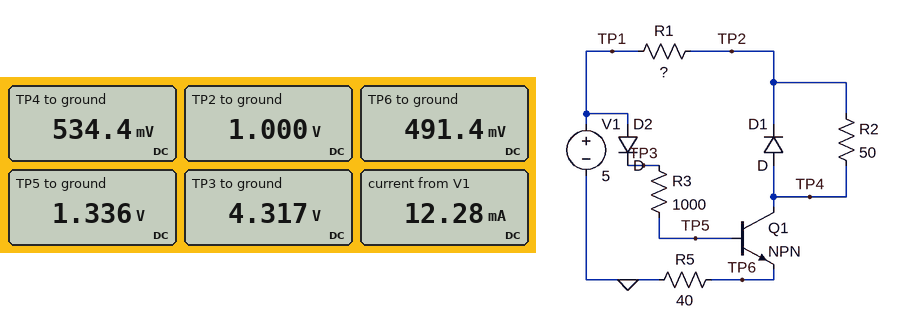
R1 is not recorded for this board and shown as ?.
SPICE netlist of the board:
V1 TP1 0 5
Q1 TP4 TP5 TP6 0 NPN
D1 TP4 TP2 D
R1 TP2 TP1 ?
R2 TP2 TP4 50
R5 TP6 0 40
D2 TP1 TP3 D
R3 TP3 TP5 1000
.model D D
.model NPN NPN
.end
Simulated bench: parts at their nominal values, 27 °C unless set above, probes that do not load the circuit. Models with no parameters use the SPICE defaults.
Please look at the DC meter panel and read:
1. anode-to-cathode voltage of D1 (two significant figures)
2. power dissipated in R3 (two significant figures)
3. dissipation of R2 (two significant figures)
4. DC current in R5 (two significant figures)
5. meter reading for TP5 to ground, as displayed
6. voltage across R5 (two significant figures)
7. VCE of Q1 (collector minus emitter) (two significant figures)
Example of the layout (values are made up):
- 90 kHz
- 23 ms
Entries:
- -470 mV
- 8.9 mW
- 4.3 mW
- 12 mA
- 1.336 V
- 490 mV
- 43 mV
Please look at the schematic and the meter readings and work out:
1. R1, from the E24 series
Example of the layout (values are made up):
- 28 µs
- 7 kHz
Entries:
- 430 Ω
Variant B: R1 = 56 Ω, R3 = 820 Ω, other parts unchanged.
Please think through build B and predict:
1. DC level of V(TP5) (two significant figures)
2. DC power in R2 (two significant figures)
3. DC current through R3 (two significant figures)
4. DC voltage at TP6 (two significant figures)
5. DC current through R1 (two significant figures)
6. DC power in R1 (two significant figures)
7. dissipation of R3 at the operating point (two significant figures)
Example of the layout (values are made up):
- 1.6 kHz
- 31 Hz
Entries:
- 2.3 V
- 55 mW
- 2.5 mA
- 1.4 V
- 33 mA
- 61 mW
- 5.0 mW
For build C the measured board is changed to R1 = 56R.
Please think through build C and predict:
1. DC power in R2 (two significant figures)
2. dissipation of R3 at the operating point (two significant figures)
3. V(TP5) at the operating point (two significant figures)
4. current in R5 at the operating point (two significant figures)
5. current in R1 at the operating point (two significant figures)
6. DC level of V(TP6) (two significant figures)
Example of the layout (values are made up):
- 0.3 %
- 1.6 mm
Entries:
- 55 mW
- 4.2 mW
- 2.3 V
- 35 mA
- 33 mA
- 1.4 V
